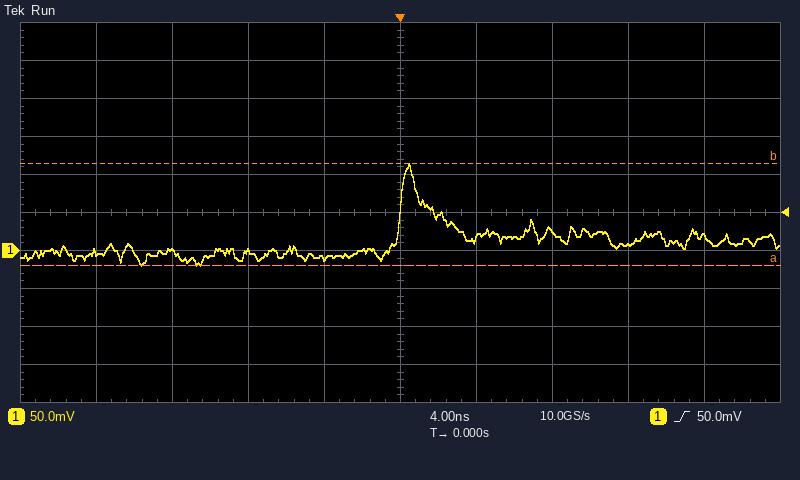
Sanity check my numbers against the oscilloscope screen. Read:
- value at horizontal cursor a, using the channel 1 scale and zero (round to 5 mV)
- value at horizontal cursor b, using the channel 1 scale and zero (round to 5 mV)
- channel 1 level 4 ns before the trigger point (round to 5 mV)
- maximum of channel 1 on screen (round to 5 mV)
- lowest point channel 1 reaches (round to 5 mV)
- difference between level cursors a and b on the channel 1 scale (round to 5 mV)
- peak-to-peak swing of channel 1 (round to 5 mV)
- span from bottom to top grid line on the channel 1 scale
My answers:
-20 mV
115 mV
-10 mV
115 mV
-20 mV
135 mV
135 mV
500 mV
